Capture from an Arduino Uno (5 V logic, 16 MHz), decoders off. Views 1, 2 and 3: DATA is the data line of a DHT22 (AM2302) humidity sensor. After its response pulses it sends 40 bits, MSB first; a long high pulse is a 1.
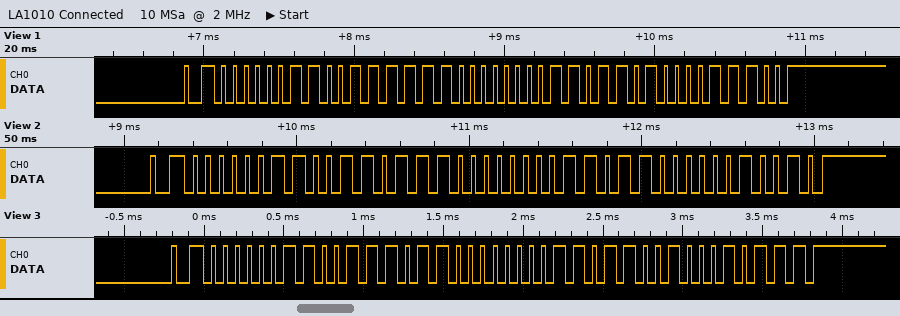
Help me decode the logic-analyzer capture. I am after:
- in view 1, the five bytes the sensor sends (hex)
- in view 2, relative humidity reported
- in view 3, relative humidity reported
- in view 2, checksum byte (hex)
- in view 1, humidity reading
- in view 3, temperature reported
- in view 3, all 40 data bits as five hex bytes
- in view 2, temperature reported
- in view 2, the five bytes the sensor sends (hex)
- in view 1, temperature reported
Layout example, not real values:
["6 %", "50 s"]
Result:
["03 3F 00 DA 1C", "82.3 %", "82.7 %", "0x12", "83.1 %", "21.7 °C", "03 3B 00 D9 17", "21.6 °C", "03 37 00 D8 12", "21.8 °C"]
